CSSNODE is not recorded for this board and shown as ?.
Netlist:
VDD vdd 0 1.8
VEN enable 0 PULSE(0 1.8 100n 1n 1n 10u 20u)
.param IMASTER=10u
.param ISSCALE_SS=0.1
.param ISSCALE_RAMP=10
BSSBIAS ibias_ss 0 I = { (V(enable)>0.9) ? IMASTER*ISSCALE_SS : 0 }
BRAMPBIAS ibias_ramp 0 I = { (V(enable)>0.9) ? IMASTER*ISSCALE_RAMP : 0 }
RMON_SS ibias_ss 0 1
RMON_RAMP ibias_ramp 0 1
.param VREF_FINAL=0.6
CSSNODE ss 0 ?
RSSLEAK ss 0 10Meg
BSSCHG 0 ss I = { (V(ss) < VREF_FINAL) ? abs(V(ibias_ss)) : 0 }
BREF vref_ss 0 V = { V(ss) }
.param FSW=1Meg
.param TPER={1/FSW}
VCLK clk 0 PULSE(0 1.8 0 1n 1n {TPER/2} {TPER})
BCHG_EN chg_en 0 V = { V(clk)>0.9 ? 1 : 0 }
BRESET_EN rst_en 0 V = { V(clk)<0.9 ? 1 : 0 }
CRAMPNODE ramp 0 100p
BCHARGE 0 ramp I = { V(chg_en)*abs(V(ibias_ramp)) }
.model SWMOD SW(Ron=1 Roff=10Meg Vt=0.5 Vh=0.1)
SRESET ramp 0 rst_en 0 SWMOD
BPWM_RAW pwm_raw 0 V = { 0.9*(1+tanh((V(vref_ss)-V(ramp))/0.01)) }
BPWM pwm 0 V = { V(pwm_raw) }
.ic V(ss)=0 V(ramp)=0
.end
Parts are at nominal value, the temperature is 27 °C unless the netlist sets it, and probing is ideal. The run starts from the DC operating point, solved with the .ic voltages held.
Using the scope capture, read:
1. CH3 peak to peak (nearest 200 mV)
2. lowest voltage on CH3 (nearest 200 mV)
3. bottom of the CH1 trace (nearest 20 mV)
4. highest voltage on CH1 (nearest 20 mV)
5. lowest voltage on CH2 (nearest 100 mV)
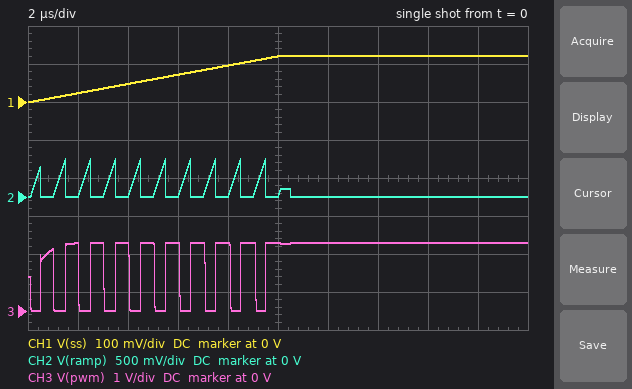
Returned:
1.8 V
0 V
0 V
120 mV
0 V
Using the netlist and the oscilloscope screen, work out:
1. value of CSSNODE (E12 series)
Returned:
82 pF
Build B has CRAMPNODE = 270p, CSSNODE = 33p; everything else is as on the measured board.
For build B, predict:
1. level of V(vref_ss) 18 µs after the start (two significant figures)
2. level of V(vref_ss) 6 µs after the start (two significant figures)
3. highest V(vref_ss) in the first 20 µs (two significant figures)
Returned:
290 mV
180 mV
300 mV
